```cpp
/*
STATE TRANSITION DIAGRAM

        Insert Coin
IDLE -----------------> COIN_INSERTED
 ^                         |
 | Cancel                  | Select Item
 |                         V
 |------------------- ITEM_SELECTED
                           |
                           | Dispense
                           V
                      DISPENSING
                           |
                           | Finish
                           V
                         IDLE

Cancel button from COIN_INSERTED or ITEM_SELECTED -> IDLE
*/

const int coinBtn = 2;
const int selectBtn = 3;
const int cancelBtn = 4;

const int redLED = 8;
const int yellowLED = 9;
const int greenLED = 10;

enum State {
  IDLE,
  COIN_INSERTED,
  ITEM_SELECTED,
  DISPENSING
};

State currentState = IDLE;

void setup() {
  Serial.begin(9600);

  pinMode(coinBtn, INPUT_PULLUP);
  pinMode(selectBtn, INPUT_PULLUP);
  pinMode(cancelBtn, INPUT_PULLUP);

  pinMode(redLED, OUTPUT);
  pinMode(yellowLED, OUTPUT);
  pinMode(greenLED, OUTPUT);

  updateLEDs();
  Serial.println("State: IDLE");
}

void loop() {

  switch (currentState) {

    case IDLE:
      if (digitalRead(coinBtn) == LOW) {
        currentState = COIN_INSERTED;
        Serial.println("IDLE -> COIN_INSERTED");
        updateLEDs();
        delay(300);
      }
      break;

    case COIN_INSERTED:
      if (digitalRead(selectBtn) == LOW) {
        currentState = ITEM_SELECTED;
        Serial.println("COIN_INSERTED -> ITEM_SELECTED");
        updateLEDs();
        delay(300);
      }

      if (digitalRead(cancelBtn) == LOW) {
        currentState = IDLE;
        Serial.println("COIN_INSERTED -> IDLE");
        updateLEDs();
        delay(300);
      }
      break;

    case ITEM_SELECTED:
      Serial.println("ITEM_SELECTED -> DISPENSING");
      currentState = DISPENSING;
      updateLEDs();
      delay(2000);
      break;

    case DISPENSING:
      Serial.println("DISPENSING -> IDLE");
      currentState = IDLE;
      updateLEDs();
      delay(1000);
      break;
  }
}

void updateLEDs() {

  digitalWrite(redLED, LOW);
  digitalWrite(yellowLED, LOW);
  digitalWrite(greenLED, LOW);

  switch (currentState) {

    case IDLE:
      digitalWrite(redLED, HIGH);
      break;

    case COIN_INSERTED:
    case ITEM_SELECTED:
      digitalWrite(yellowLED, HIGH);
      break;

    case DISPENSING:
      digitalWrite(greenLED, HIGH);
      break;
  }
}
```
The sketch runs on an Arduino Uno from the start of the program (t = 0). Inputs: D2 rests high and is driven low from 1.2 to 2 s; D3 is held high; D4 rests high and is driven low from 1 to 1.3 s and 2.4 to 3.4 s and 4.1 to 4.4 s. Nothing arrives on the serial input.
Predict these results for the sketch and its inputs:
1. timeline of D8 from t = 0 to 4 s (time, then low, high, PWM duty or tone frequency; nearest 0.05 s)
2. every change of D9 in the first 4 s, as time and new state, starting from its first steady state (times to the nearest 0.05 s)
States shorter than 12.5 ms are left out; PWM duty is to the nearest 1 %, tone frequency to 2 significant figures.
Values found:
0 s high; 1.2 s low; 2.4 s high
0 s low; 1.2 s high; 2.4 s low
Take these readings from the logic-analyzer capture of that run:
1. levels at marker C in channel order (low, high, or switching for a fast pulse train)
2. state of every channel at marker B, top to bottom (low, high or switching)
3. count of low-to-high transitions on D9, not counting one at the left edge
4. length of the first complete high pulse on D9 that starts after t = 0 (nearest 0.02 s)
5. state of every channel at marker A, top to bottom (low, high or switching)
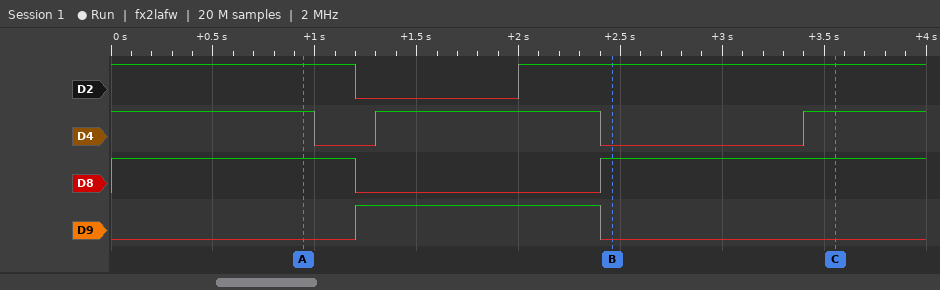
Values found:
D2 high, D4 high, D8 high, D9 low
D2 high, D4 low, D8 high, D9 low
1
1.20 s
D2 high, D4 high, D8 high, D9 low
